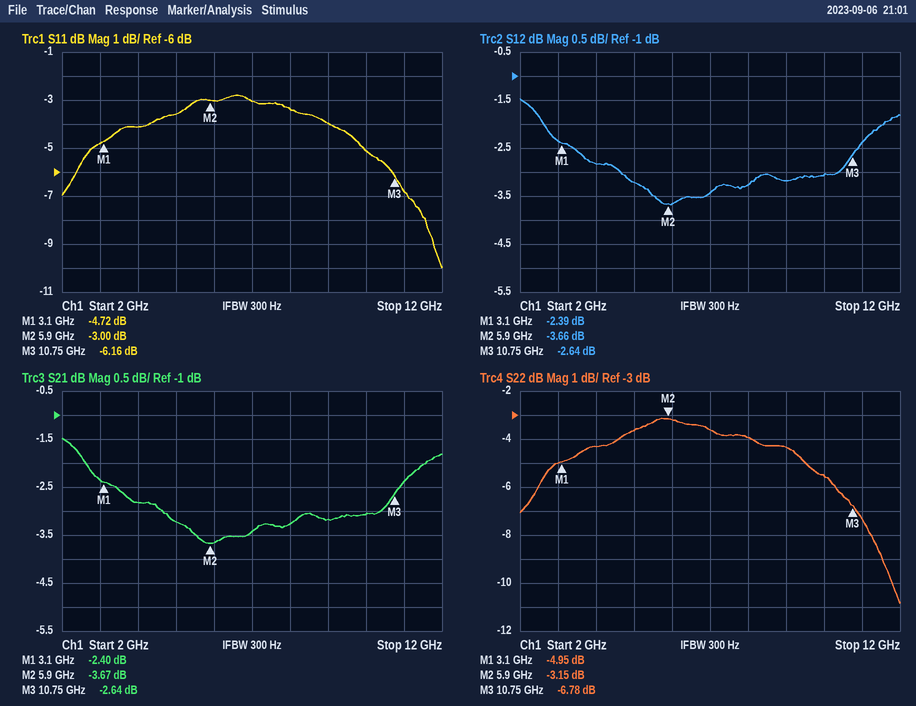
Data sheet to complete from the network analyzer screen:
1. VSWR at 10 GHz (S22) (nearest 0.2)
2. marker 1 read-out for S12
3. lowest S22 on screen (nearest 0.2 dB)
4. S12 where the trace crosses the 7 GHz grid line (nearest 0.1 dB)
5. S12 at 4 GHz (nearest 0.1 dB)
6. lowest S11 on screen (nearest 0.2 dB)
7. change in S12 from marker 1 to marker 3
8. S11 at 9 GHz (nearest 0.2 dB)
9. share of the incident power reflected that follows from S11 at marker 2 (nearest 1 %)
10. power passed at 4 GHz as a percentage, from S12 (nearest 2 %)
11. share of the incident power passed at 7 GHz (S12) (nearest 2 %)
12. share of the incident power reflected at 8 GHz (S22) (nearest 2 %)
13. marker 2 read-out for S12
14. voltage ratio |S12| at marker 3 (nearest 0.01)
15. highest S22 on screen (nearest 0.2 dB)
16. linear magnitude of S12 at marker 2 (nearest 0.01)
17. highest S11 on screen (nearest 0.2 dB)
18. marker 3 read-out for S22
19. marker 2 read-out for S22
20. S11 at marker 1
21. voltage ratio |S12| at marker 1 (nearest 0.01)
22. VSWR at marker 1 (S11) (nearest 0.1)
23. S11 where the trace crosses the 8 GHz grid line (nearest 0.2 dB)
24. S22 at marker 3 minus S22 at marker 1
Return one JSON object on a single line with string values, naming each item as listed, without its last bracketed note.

{"VSWR at 10 GHz (S22)": "3.2", "marker 1 read-out for S12": "-2.39 dB", "lowest S22 on screen": "-10.8 dB", "S12 where the trace crosses the 7 GHz grid line": "-3.4 dB", "S12 at 4 GHz": "-2.8 dB", "lowest S11 on screen": "-10.0 dB", "change in S12 from marker 1 to marker 3": "-0.25 dB", "S11 at 9 GHz": "-4.0 dB", "share of the incident power reflected that follows from S11 at marker 2": "50 %", "power passed at 4 GHz as a percentage, from S12": "52 %", "share of the incident power passed at 7 GHz (S12)": "46 %", "share of the incident power reflected at 8 GHz (S22)": "40 %", "marker 2 read-out for S12": "-3.66 dB", "voltage ratio |S12| at marker 3": "0.74", "highest S22 on screen": "-3.2 dB", "linear magnitude of S12 at marker 2": "0.66", "highest S11 on screen": "-2.8 dB", "marker 3 read-out for S22": "-6.78 dB", "marker 2 read-out for S22": "-3.15 dB", "S11 at marker 1": "-4.72 dB", "voltage ratio |S12| at marker 1": "0.76", "VSWR at marker 1 (S11)": "3.8", "S11 where the trace crosses the 8 GHz grid line": "-3.4 dB", "S22 at marker 3 minus S22 at marker 1": "-1.83 dB"}
